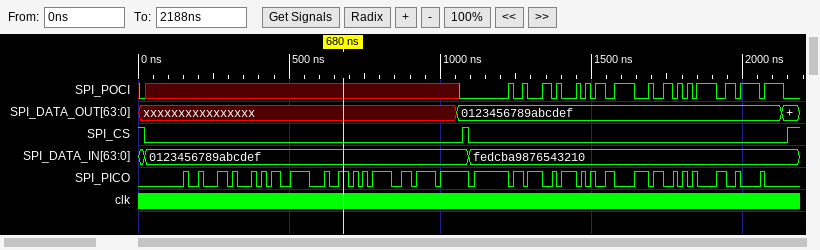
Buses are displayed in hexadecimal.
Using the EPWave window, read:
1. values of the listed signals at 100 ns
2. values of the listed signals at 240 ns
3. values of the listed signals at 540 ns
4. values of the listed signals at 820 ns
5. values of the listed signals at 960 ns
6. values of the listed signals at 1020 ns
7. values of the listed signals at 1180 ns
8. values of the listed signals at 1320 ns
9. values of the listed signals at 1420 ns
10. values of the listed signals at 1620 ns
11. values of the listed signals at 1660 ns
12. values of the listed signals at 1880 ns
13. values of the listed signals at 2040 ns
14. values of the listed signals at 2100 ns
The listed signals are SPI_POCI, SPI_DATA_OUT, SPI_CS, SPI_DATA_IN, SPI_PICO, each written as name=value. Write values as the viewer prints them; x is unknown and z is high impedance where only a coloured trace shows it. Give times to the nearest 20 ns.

SPI_POCI=x, SPI_DATA_OUT=xxxxxxxxxxxxxxxx, SPI_CS=0, SPI_DATA_IN=0123456789abcdef, SPI_PICO=0
SPI_POCI=x, SPI_DATA_OUT=xxxxxxxxxxxxxxxx, SPI_CS=0, SPI_DATA_IN=0123456789abcdef, SPI_PICO=0
SPI_POCI=x, SPI_DATA_OUT=xxxxxxxxxxxxxxxx, SPI_CS=0, SPI_DATA_IN=0123456789abcdef, SPI_PICO=1
SPI_POCI=x, SPI_DATA_OUT=xxxxxxxxxxxxxxxx, SPI_CS=0, SPI_DATA_IN=0123456789abcdef, SPI_PICO=1
SPI_POCI=x, SPI_DATA_OUT=xxxxxxxxxxxxxxxx, SPI_CS=0, SPI_DATA_IN=0123456789abcdef, SPI_PICO=1
SPI_POCI=x, SPI_DATA_OUT=xxxxxxxxxxxxxxxx, SPI_CS=0, SPI_DATA_IN=0123456789abcdef, SPI_PICO=1
SPI_POCI=0, SPI_DATA_OUT=0123456789abcdef, SPI_CS=0, SPI_DATA_IN=fedcba9876543210, SPI_PICO=1
SPI_POCI=0, SPI_DATA_OUT=0123456789abcdef, SPI_CS=0, SPI_DATA_IN=fedcba9876543210, SPI_PICO=1
SPI_POCI=0, SPI_DATA_OUT=0123456789abcdef, SPI_CS=0, SPI_DATA_IN=fedcba9876543210, SPI_PICO=1
SPI_POCI=1, SPI_DATA_OUT=0123456789abcdef, SPI_CS=0, SPI_DATA_IN=fedcba9876543210, SPI_PICO=0
SPI_POCI=0, SPI_DATA_OUT=0123456789abcdef, SPI_CS=0, SPI_DATA_IN=fedcba9876543210, SPI_PICO=1
SPI_POCI=1, SPI_DATA_OUT=0123456789abcdef, SPI_CS=0, SPI_DATA_IN=fedcba9876543210, SPI_PICO=0
SPI_POCI=1, SPI_DATA_OUT=0123456789abcdef, SPI_CS=0, SPI_DATA_IN=fedcba9876543210, SPI_PICO=0
SPI_POCI=1, SPI_DATA_OUT=0123456789abcdef, SPI_CS=0, SPI_DATA_IN=fedcba9876543210, SPI_PICO=0
